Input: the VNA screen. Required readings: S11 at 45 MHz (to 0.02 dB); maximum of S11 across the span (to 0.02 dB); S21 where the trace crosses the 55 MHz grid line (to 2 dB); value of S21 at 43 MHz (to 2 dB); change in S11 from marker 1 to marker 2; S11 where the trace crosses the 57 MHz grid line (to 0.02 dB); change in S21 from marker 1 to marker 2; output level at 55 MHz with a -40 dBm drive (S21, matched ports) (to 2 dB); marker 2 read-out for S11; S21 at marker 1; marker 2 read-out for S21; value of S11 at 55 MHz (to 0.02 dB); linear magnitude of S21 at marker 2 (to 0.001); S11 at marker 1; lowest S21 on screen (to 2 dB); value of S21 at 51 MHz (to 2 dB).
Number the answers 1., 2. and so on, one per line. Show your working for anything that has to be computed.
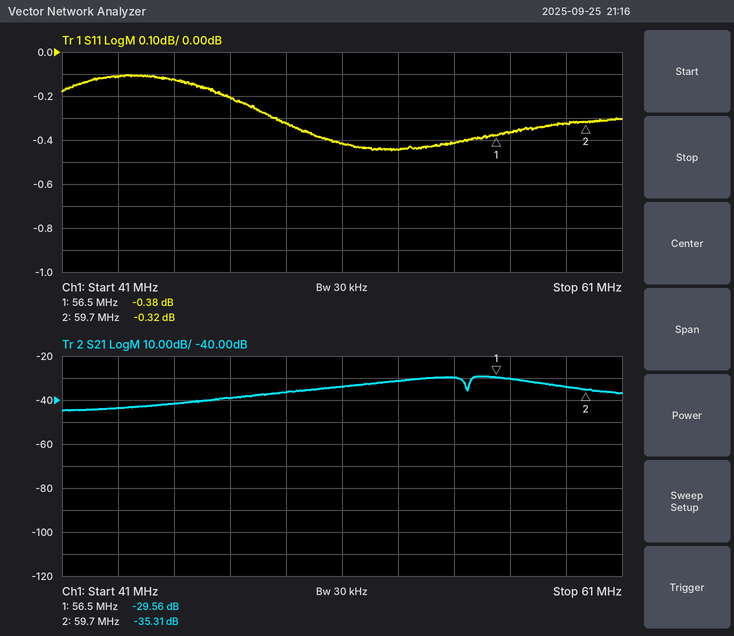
1. -0.12 dB
2. -0.10 dB
3. -30 dB
4. -44 dB
5. -0.32 − (-0.38) = 0.06 dB
6. -0.36 dB
7. -35.31 − (-29.56) = -5.75 dB
8. -40 dBm + (-30 dB) = -70 dBm
9. -0.32 dB
10. -29.56 dB
11. -35.31 dB
12. -0.42 dB
13. 10^(-35.31/20) ≈ 0.017
14. -0.38 dB
15. -44 dB
16. -34 dB
